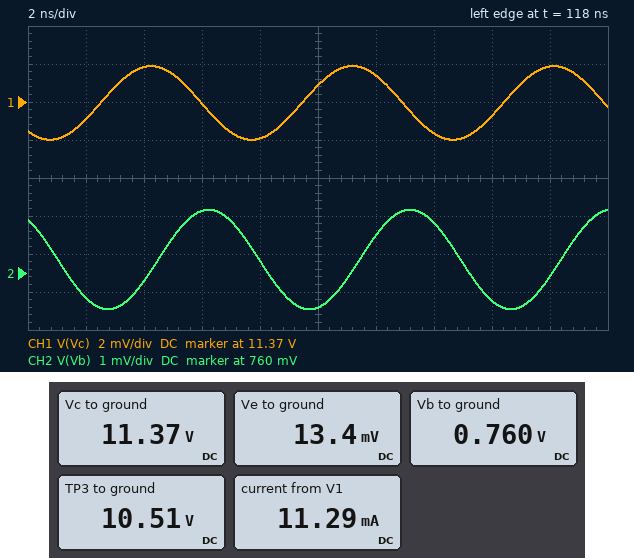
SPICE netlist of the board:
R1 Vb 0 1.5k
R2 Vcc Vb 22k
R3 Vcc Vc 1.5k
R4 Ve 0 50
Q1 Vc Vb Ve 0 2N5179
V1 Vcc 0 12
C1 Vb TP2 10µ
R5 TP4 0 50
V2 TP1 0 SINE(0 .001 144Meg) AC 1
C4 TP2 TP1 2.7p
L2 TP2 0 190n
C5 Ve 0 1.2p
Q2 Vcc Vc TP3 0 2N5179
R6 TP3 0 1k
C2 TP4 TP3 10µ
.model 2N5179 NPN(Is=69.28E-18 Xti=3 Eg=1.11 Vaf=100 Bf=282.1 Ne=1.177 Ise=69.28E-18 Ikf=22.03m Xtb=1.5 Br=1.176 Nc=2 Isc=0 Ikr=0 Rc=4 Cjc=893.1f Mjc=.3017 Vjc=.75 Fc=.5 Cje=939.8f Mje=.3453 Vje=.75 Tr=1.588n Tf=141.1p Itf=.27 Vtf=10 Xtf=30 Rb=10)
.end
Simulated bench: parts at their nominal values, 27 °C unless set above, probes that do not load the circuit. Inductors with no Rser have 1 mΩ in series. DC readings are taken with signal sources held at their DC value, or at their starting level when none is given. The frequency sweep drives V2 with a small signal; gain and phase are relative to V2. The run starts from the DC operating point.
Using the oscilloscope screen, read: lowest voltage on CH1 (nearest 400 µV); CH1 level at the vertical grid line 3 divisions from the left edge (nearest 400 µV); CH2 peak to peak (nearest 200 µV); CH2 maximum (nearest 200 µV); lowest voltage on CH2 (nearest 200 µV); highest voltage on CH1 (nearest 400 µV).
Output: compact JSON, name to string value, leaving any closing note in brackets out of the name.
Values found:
{"lowest voltage on CH1": "11.3640 V", "CH1 level at the vertical grid line 3 divisions from the left edge": "11.3660 V", "CH2 peak to peak": "2.6 mV", "CH2 maximum": "761.6 mV", "lowest voltage on CH2": "759.0 mV", "highest voltage on CH1": "11.3680 V"}
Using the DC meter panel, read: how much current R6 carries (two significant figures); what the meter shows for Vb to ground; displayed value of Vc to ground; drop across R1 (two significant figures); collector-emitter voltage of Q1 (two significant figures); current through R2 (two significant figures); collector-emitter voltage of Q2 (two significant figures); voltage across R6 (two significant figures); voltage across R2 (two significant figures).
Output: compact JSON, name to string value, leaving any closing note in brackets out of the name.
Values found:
{"how much current R6 carries": "11 mA", "what the meter shows for Vb to ground": "0.760 V", "displayed value of Vc to ground": "11.37 V", "drop across R1": "760 mV", "collector-emitter voltage of Q1": "11 V", "current through R2": "510 µA", "collector-emitter voltage of Q2": "1.5 V", "voltage across R6": "11 V", "voltage across R2": "11 V"}
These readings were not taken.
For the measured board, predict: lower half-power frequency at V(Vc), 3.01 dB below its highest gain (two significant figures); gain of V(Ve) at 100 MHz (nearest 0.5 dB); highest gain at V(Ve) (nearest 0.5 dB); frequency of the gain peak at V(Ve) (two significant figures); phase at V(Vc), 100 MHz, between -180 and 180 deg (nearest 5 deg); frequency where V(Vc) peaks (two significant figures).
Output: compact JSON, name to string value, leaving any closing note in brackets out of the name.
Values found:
{"lower half-power frequency at V(Vc), 3.01 dB below its highest gain": "140 MHz", "gain of V(Ve) at 100 MHz": "-19.0 dB", "highest gain at V(Ve)": "-4.0 dB", "frequency of the gain peak at V(Ve)": "160 MHz", "phase at V(Vc), 100 MHz, between -180 and 180 deg": "-85 deg", "frequency where V(Vc) peaks": "160 MHz"}
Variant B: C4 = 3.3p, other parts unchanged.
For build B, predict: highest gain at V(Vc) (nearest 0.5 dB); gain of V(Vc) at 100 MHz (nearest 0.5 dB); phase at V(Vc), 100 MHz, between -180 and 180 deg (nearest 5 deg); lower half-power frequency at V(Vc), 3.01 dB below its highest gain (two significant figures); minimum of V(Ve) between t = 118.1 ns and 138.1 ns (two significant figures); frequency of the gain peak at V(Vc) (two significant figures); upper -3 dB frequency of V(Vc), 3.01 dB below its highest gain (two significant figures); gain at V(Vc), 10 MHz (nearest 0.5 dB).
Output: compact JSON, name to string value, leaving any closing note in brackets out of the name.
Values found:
{"highest gain at V(Vc)": "9.5 dB", "gain of V(Vc) at 100 MHz": "-1.0 dB", "phase at V(Vc), 100 MHz, between -180 and 180 deg": "-90 deg", "lower half-power frequency at V(Vc), 3.01 dB below its highest gain": "130 MHz", "minimum of V(Ve) between t = 118.1 ns and 138.1 ns": "13 mV", "frequency of the gain peak at V(Vc)": "150 MHz", "upper -3 dB frequency of V(Vc), 3.01 dB below its highest gain": "170 MHz", "gain at V(Vc), 10 MHz": "-36.0 dB"}
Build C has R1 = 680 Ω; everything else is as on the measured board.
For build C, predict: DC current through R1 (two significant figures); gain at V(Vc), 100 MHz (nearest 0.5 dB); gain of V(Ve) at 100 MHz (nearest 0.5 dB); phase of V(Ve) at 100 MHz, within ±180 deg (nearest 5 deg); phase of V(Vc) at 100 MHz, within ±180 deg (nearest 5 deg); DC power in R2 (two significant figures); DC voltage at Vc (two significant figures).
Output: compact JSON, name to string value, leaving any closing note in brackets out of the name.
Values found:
{"DC current through R1": "530 µA", "gain at V(Vc), 100 MHz": "-33.5 dB", "gain of V(Ve) at 100 MHz": "-39.5 dB", "phase of V(Ve) at 100 MHz, within ±180 deg": "-110 deg", "phase of V(Vc) at 100 MHz, within ±180 deg": "-170 deg", "DC power in R2": "6.2 mW", "DC voltage at Vc": "12 V"}
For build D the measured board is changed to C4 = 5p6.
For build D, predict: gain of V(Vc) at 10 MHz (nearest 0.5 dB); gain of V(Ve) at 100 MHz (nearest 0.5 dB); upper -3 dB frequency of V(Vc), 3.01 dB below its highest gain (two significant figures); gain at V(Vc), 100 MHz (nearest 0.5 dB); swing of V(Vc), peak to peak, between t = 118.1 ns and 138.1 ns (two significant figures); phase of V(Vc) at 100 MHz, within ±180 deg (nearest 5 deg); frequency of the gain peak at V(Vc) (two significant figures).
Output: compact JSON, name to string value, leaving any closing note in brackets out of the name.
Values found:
{"gain of V(Vc) at 10 MHz": "-31.5 dB", "gain of V(Ve) at 100 MHz": "-9.5 dB", "upper -3 dB frequency of V(Vc), 3.01 dB below its highest gain": "140 MHz", "gain at V(Vc), 100 MHz": "6.5 dB", "swing of V(Vc), peak to peak, between t = 118.1 ns and 138.1 ns": "7.1 mV", "phase of V(Vc) at 100 MHz, within ±180 deg": "-95 deg", "frequency of the gain peak at V(Vc)": "130 MHz"}
